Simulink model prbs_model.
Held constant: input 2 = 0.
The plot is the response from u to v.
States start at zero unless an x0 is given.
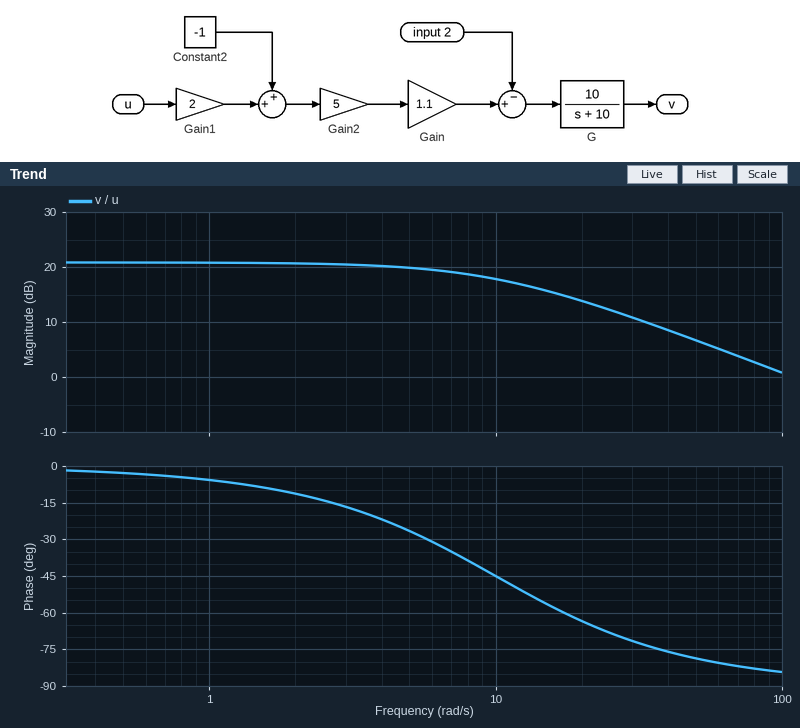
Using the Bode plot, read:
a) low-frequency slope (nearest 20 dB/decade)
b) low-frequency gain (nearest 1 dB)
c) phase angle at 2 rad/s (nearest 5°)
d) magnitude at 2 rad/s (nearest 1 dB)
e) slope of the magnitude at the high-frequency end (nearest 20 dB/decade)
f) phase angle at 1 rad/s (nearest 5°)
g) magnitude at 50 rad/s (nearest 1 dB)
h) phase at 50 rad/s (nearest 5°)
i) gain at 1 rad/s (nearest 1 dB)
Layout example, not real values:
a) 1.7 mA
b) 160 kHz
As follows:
a) 0 dB/decade
b) 21 dB
c) -10°
d) 21 dB
e) -20 dB/decade
f) -5°
g) 7 dB
h) -80°
i) 21 dB
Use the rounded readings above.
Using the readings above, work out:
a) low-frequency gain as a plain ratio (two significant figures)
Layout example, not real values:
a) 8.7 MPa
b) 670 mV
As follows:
a) 11
